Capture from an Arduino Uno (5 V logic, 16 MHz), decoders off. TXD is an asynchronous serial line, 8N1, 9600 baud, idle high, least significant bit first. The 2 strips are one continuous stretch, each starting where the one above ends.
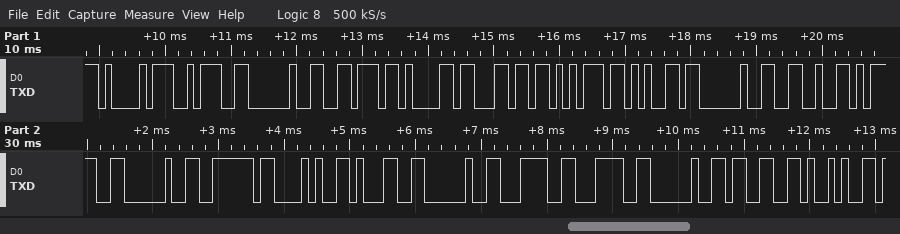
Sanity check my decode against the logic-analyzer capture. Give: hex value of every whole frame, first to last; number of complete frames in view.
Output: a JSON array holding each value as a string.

["0xA1 0x3A 0x20 0x76 0x61 0x6C 0x75 0x65 0x20 0x26 0x3D 0x20 0x7E 0x28 0x31 0x20 0x3C 0x3C 0x20 0x33 0x29", "21"]
